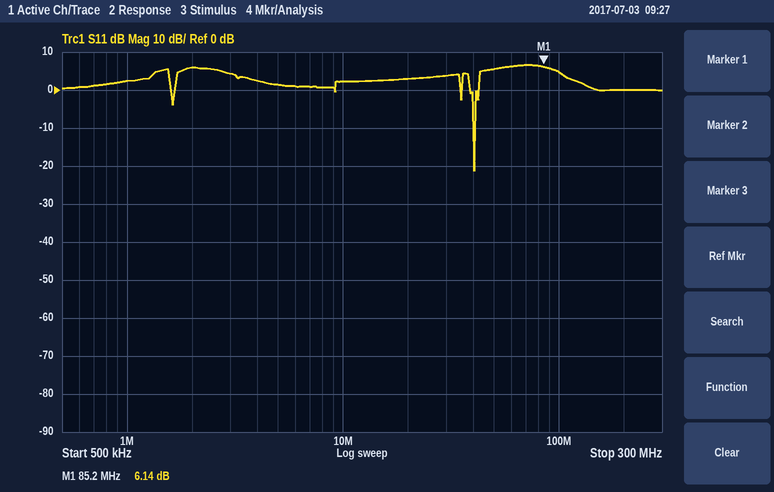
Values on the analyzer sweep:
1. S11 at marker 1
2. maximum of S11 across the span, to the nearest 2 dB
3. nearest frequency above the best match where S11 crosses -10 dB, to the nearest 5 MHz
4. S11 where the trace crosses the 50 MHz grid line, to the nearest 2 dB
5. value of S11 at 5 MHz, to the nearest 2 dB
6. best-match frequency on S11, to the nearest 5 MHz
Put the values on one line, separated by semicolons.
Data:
6.14 dB; 6 dB; 40 MHz; 6 dB; 2 dB; 40 MHz
